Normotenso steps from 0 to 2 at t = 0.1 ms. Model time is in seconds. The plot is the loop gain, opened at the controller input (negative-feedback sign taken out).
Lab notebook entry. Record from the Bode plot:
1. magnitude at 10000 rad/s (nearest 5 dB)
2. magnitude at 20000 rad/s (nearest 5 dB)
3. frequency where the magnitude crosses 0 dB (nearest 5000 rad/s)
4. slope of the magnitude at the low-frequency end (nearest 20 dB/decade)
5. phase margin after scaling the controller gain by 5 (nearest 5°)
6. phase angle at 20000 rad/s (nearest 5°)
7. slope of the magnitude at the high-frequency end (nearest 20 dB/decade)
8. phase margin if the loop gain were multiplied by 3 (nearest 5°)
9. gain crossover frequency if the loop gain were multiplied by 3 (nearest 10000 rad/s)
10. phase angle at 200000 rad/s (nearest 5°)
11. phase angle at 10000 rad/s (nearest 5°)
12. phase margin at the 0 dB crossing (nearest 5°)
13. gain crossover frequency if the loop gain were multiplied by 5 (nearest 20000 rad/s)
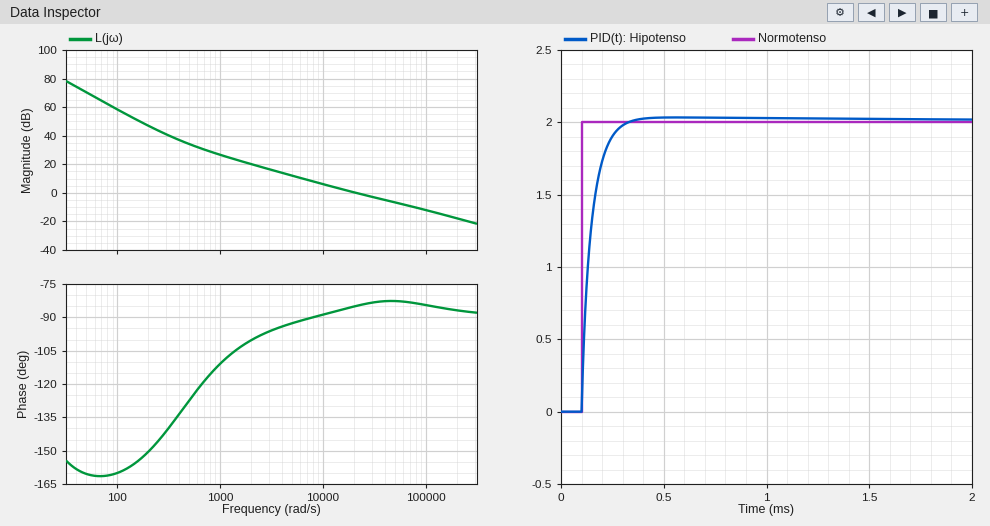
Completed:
5 dB
0 dB
20000 rad/s
-40 dB/decade
95°
-85°
-20 dB/decade
95°
70000 rad/s
-85°
-90°
95°
120000 rad/s
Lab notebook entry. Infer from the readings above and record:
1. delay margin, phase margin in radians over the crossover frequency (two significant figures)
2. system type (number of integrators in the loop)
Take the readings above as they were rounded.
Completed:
0.000083 s
2
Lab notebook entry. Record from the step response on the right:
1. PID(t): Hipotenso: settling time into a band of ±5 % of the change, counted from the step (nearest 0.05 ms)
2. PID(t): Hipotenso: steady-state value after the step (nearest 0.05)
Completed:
0.15 ms
2.00
